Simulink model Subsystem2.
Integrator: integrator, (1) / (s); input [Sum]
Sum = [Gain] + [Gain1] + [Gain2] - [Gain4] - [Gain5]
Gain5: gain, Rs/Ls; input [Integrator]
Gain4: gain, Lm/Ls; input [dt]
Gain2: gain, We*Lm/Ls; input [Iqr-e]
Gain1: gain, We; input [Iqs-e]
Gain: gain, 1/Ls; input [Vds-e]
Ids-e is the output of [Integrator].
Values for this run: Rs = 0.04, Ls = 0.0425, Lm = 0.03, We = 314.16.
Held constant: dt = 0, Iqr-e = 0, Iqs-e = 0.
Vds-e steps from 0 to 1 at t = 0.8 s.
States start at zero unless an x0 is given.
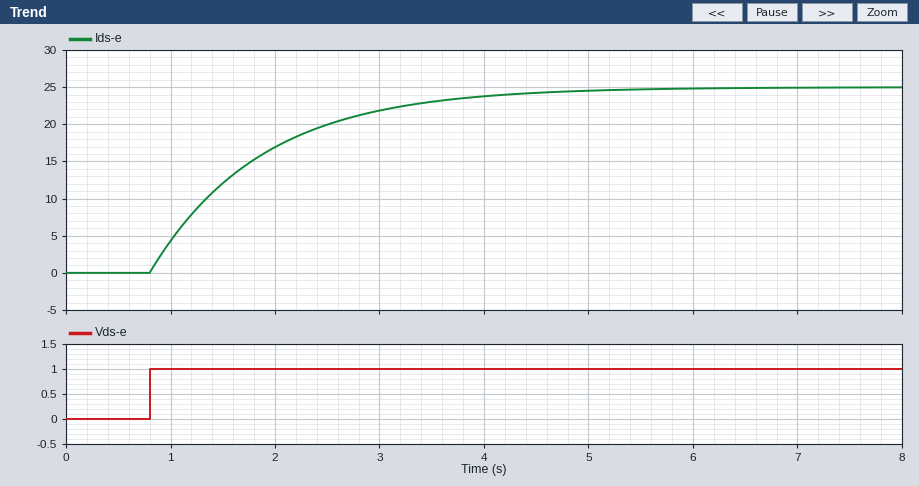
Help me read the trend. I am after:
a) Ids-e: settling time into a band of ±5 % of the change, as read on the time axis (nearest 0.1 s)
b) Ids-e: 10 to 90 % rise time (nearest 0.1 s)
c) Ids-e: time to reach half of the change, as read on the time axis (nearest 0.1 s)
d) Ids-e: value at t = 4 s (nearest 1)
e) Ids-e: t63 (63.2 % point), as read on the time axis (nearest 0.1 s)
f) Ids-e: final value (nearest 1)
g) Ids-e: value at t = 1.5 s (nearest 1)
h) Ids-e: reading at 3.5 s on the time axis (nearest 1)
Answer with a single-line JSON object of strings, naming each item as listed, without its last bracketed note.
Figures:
{"Ids-e: settling time into a band of ±5 % of the change, as read on the time axis": "4.0 s", "Ids-e: 10 to 90 % rise time": "2.3 s", "Ids-e: time to reach half of the change, as read on the time axis": "1.5 s", "Ids-e: value at t = 4 s": "24", "Ids-e: t63 (63.2 % point), as read on the time axis": "1.9 s", "Ids-e: final value": "25", "Ids-e: value at t = 1.5 s": "12", "Ids-e: reading at 3.5 s on the time axis": "23"}
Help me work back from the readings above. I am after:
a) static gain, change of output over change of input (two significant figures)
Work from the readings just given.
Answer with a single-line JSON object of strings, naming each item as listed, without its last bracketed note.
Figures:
{"static gain, change of output over change of input": "25"}
